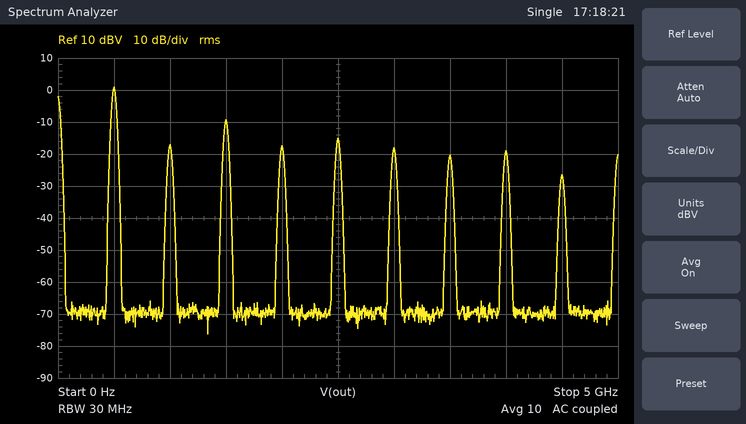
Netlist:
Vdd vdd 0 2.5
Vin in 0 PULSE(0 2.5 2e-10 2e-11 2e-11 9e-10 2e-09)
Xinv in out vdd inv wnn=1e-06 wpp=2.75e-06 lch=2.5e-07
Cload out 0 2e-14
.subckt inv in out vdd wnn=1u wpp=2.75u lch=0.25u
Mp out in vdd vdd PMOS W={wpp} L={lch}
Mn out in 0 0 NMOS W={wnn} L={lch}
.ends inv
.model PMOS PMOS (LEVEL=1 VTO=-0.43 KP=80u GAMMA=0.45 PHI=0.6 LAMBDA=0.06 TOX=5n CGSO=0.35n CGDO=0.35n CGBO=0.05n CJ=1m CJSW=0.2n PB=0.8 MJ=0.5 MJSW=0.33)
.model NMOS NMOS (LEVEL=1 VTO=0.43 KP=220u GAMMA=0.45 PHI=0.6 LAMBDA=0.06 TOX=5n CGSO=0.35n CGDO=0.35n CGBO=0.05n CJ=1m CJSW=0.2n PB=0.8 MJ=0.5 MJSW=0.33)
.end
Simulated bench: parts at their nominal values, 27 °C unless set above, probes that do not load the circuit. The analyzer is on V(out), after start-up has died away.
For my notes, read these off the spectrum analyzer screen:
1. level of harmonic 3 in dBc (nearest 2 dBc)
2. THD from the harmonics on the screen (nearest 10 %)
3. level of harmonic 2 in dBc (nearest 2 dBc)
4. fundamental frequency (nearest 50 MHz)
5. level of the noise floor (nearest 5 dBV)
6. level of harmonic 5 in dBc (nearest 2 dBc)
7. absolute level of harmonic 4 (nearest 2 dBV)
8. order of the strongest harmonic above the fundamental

-10 dBc
40 %
-18 dBc
500 MHz
-70 dBV
-16 dBc
-18 dBV
3
